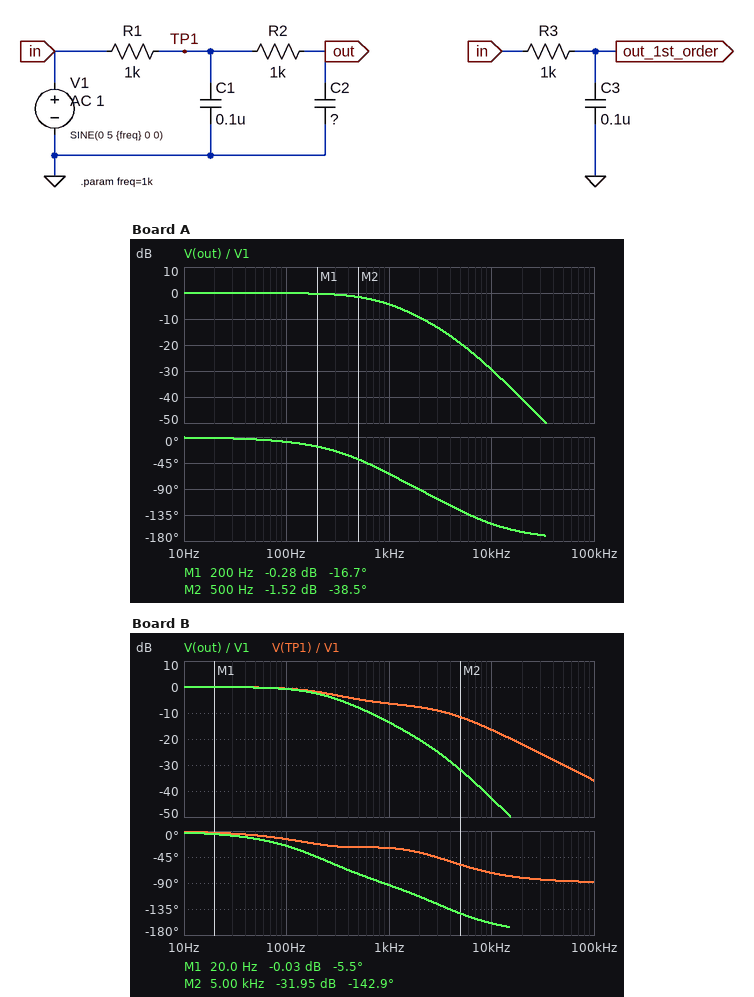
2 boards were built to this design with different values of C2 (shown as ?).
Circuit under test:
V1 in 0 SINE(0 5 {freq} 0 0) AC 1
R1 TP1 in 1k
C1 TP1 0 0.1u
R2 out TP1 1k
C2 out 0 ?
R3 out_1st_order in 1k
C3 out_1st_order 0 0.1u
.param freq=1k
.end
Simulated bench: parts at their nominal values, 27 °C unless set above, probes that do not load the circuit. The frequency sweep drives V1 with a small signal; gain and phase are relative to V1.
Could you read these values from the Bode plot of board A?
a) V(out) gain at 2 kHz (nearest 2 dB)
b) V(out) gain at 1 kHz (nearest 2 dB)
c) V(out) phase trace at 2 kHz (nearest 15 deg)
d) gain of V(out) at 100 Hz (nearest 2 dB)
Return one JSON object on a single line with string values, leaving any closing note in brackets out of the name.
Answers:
{"V(out) gain at 2 kHz": "-10 dB", "V(out) gain at 1 kHz": "-4 dB", "V(out) phase trace at 2 kHz": "-90 deg", "gain of V(out) at 100 Hz": "0 dB"}
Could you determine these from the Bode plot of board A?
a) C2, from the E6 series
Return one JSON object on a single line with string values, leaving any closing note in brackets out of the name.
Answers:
{"C2, from the E6 series": "68 nF"}
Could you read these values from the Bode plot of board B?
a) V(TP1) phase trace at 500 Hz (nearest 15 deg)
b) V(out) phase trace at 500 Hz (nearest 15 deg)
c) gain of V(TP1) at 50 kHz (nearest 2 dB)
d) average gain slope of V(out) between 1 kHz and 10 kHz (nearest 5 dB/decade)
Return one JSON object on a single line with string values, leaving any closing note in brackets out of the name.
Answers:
{"V(TP1) phase trace at 500 Hz": "-30 deg", "V(out) phase trace at 500 Hz": "-75 deg", "gain of V(TP1) at 50 kHz": "-30 dB", "average gain slope of V(out) between 1 kHz and 10 kHz": "-30 dB/decade"}
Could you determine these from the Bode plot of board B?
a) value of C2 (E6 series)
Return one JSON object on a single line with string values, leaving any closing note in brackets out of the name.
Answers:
{"value of C2": "330 nF"}
